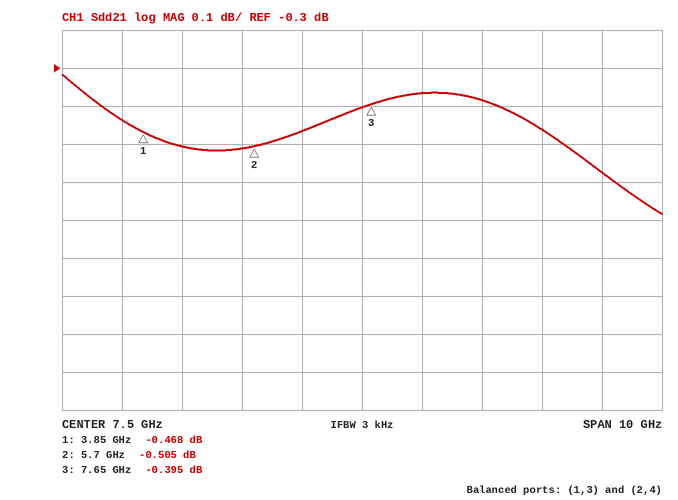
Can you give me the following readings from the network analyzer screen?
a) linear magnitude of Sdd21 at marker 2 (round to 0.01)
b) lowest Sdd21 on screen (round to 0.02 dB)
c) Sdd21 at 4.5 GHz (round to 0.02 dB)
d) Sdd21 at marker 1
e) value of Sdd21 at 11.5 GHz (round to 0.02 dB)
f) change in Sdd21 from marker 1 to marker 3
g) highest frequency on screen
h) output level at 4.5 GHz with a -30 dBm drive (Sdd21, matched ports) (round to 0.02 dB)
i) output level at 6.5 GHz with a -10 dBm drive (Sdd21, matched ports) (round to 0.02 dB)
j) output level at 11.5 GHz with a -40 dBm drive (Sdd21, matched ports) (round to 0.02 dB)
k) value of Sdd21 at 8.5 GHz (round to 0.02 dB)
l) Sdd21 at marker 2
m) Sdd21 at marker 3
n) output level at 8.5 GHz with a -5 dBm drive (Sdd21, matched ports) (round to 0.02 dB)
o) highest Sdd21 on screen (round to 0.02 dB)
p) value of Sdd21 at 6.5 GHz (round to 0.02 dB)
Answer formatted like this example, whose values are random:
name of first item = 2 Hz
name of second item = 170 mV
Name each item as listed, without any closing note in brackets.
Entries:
linear magnitude of Sdd21 at marker 2 = 0.94
lowest Sdd21 on screen = -0.68 dB
Sdd21 at 4.5 GHz = -0.50 dB
Sdd21 at marker 1 = -0.468 dB
value of Sdd21 at 11.5 GHz = -0.58 dB
change in Sdd21 from marker 1 to marker 3 = 0.073 dB
highest frequency on screen = 12.5 GHz
output level at 4.5 GHz with a -30 dBm drive (Sdd21, matched ports) = -30.50 dBm
output level at 6.5 GHz with a -10 dBm drive (Sdd21, matched ports) = -10.46 dBm
output level at 11.5 GHz with a -40 dBm drive (Sdd21, matched ports) = -40.58 dBm
value of Sdd21 at 8.5 GHz = -0.36 dB
Sdd21 at marker 2 = -0.505 dB
Sdd21 at marker 3 = -0.395 dB
output level at 8.5 GHz with a -5 dBm drive (Sdd21, matched ports) = -5.36 dBm
highest Sdd21 on screen = -0.32 dB
value of Sdd21 at 6.5 GHz = -0.46 dB
